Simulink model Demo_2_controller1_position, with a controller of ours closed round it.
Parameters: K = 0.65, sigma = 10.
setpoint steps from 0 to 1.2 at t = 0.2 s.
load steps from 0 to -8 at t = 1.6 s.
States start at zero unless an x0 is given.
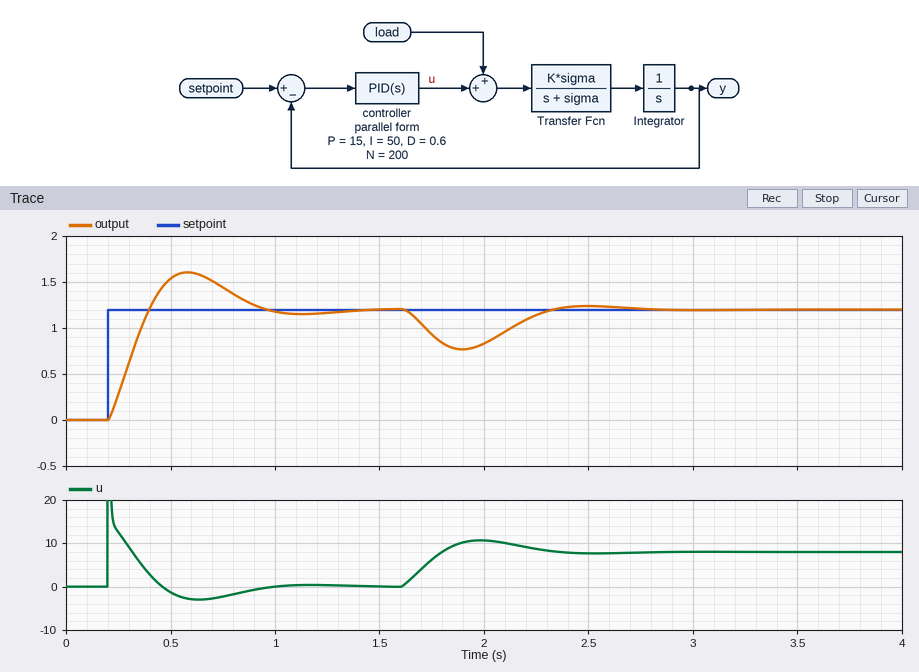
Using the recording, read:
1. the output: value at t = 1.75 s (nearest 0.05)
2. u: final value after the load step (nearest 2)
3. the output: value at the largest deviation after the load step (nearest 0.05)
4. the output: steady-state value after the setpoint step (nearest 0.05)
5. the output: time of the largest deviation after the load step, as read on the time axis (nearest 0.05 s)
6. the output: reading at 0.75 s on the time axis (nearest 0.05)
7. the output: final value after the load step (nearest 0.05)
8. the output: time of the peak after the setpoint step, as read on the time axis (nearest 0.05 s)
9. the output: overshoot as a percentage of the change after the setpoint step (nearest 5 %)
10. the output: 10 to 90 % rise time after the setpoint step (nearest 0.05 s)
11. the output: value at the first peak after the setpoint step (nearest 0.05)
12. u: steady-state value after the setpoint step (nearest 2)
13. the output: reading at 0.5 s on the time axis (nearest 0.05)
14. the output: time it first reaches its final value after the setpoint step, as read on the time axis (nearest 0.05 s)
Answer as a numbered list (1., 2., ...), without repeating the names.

1. 0.95
2. 8
3. 0.75
4. 1.20
5. 1.90 s
6. 1.45
7. 1.20
8. 0.60 s
9. 35 %
10. 0.15 s
11. 1.60
12. 0
13. 1.55
14. 0.40 s
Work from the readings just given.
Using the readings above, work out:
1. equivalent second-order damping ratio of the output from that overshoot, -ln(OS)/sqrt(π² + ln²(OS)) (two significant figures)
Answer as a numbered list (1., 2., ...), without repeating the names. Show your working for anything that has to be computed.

1. ln(0.35) = -1.050; 1.050 / sqrt(9.870 + 1.102) = 0.32
